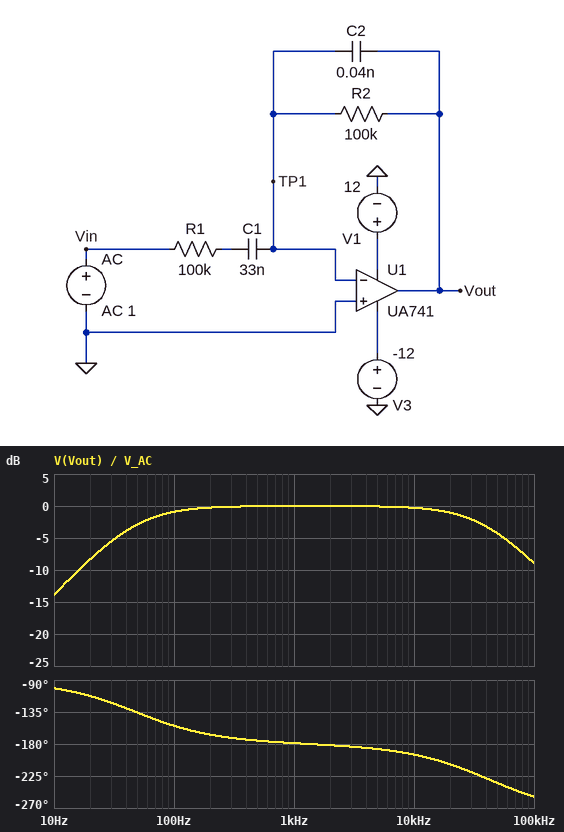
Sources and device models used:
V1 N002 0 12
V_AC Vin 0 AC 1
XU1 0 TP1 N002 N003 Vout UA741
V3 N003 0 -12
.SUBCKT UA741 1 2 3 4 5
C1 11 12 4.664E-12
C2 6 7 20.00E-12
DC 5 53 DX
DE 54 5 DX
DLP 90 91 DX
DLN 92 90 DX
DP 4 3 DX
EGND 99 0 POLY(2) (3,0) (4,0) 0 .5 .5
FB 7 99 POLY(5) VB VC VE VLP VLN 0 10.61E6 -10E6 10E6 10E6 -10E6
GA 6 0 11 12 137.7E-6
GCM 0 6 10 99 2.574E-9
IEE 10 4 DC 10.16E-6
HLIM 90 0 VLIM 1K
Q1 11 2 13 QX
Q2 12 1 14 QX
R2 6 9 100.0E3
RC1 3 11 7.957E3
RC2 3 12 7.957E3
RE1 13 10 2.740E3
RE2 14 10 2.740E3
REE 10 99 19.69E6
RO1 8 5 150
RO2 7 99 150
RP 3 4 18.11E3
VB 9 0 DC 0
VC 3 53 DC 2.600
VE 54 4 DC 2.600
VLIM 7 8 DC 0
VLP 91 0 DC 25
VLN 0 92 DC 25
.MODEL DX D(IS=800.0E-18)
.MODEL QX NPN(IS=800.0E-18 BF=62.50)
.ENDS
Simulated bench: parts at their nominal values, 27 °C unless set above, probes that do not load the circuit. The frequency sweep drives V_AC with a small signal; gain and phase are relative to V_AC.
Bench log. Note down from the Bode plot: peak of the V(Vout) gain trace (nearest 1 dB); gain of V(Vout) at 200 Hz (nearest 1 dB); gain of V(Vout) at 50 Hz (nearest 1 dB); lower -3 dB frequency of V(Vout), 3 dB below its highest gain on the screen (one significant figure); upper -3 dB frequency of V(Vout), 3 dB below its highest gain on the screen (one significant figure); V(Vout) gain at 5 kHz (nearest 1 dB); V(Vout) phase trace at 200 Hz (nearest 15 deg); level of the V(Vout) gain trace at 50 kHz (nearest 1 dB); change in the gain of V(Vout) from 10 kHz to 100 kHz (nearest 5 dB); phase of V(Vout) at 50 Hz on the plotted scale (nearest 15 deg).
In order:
0 dB
0 dB
-3 dB
50 Hz
40 kHz
0 dB
-165 deg
-4 dB
-10 dB
-135 deg
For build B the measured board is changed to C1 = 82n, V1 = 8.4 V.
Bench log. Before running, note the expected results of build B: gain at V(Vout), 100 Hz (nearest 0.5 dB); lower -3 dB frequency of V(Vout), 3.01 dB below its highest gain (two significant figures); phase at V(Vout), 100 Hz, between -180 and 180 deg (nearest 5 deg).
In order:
0 dB
19 Hz
-170 deg
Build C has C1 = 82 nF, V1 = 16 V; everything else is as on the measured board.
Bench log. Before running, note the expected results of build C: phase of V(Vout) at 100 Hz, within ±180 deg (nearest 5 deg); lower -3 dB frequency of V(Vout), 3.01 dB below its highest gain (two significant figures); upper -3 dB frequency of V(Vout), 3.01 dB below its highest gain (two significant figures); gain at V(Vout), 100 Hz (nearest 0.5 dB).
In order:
-170 deg
19 Hz
38 kHz
0 dB
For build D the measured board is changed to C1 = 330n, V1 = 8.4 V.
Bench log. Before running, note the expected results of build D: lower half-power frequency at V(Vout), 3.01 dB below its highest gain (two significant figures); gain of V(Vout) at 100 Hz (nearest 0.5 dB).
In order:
4.8 Hz
0 dB
